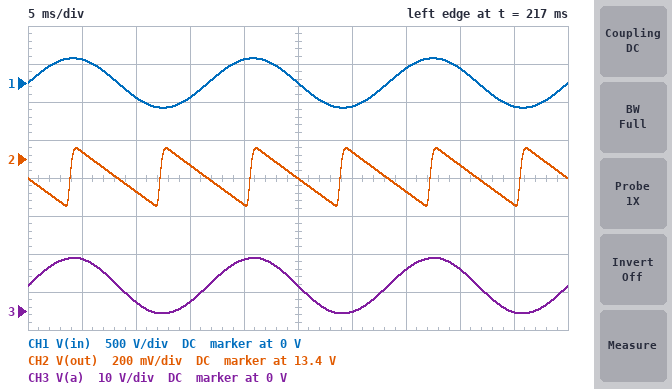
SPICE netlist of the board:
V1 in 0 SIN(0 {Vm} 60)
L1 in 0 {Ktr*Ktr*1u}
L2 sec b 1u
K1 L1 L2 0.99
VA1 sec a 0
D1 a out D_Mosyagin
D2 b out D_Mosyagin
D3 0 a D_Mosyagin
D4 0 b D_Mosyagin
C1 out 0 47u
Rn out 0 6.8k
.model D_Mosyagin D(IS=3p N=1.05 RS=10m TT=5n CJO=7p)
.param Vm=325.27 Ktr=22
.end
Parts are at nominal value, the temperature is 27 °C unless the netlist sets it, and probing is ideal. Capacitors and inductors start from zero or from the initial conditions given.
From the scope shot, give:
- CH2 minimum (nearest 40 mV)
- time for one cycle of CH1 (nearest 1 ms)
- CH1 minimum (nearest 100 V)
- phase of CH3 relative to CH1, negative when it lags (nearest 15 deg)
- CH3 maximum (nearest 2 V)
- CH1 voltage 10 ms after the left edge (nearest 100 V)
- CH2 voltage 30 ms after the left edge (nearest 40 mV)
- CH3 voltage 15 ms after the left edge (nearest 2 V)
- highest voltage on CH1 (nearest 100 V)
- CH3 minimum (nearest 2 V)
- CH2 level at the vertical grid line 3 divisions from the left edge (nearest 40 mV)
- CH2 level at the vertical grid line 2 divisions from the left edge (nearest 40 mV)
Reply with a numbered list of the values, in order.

1. 13.16 V
2. 17 ms
3. -300 V
4. 0 deg
5. 14 V
6. -200 V
7. 13.44 V
8. 2 V
9. 300 V
10. 0 V
11. 13.36 V
12. 13.24 V
